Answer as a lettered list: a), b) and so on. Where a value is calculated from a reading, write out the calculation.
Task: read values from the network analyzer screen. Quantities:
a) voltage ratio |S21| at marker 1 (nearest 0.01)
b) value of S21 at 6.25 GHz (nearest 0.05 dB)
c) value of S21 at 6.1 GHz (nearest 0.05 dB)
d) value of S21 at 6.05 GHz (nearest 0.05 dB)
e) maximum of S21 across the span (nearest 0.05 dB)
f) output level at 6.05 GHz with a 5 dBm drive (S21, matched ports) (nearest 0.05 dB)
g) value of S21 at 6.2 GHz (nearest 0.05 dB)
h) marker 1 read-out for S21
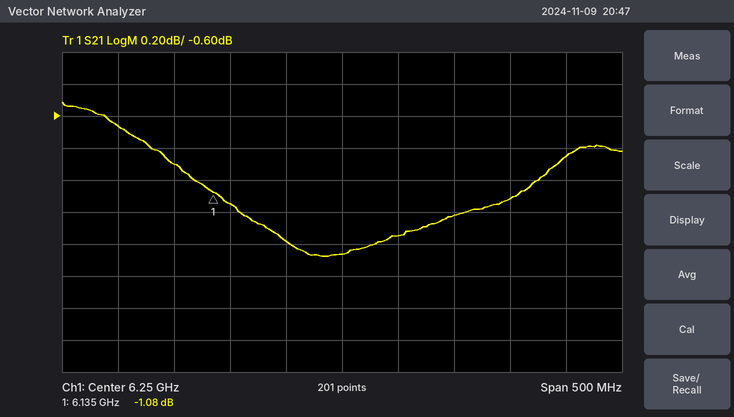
a) 10^(-1.08/20) ≈ 0.88
b) -1.45 dB
c) -0.90 dB
d) -0.65 dB
e) -0.50 dB
f) 5 dBm + (-0.65 dB) = 4.35 dBm
g) -1.40 dB
h) -1.08 dB
